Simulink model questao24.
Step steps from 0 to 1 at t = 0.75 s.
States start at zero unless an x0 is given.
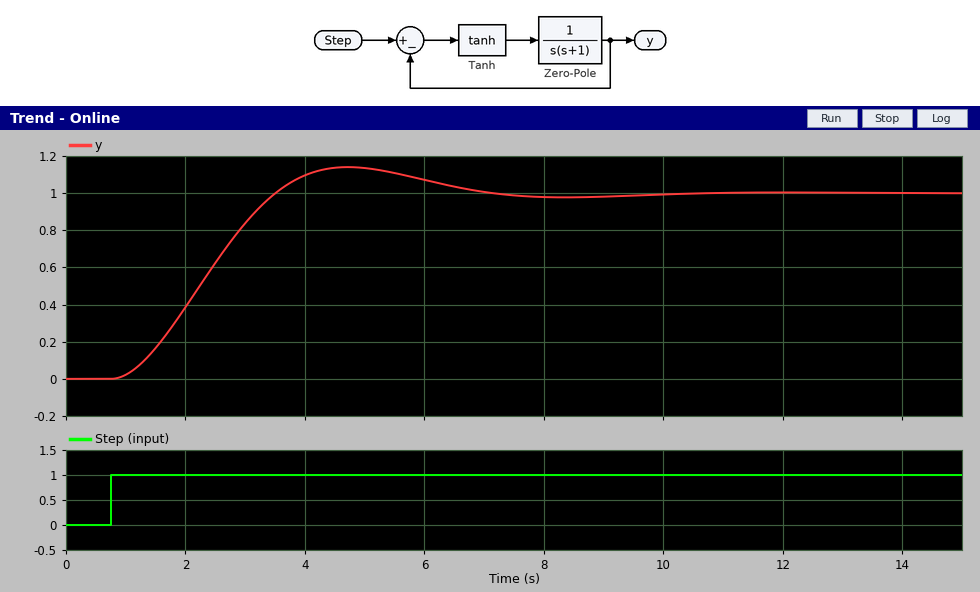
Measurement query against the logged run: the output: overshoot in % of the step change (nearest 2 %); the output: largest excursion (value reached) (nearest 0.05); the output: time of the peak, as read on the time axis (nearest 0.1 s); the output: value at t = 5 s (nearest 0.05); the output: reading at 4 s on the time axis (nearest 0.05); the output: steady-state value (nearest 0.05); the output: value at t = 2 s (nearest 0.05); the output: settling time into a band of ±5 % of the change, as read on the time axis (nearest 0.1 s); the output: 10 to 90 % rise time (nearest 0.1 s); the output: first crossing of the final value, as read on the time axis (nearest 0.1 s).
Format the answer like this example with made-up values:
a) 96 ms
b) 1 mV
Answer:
a) 14 %
b) 1.15
c) 4.7 s
d) 1.15
e) 1.10
f) 1.00
g) 0.40
h) 6.3 s
i) 1.9 s
j) 3.5 s
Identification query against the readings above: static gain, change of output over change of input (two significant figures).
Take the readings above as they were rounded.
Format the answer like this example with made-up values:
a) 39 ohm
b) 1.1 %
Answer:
a) 1.0
